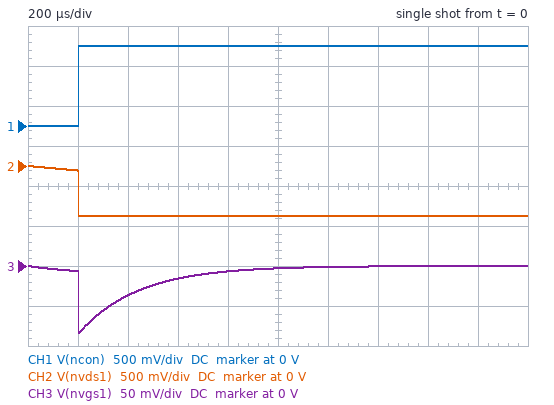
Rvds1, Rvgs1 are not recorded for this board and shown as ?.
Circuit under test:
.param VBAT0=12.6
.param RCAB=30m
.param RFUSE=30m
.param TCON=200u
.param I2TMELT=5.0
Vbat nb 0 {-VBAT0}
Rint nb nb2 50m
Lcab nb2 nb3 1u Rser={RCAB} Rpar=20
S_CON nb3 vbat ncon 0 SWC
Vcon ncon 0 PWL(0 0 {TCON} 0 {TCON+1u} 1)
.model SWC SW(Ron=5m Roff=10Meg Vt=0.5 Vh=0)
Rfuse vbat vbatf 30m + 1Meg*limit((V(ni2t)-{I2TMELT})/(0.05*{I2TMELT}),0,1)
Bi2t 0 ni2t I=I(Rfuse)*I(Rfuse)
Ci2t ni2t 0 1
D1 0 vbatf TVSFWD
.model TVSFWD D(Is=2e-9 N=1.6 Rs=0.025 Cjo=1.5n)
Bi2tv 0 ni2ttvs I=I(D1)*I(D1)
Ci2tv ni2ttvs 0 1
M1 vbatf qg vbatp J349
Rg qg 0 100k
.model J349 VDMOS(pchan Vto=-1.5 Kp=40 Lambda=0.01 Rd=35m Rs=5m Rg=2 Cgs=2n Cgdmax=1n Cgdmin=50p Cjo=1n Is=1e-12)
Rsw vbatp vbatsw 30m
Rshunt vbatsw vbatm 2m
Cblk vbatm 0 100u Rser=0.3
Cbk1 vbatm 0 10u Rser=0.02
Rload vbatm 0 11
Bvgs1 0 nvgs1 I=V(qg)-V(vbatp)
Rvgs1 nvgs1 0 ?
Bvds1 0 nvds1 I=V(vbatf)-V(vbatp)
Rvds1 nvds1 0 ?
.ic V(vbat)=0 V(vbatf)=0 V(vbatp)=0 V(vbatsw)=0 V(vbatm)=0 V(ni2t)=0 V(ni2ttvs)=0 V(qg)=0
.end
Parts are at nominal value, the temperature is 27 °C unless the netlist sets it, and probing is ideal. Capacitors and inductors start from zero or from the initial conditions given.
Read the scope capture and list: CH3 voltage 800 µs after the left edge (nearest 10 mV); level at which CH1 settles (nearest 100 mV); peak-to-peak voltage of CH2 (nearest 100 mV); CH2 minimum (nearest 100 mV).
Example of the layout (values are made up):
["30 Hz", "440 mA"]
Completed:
["-10 mV", "1.0 V", "600 mV", "-600 mV"]
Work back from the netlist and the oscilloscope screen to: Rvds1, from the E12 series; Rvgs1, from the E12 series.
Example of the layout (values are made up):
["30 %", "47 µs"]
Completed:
["0.68 Ω", "0.47 Ω"]
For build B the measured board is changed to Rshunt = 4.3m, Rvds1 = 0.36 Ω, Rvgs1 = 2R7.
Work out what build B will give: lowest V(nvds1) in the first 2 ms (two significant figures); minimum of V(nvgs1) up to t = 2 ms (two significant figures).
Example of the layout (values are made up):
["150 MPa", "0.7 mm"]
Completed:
["-330 mV", "-480 mV"]
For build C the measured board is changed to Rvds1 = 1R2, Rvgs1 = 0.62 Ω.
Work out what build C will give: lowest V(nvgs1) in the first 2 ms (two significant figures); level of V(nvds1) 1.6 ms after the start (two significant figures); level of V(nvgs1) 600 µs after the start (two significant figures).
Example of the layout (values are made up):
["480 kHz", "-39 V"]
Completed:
["-110 mV", "-1.1 V", "-21 mV"]
